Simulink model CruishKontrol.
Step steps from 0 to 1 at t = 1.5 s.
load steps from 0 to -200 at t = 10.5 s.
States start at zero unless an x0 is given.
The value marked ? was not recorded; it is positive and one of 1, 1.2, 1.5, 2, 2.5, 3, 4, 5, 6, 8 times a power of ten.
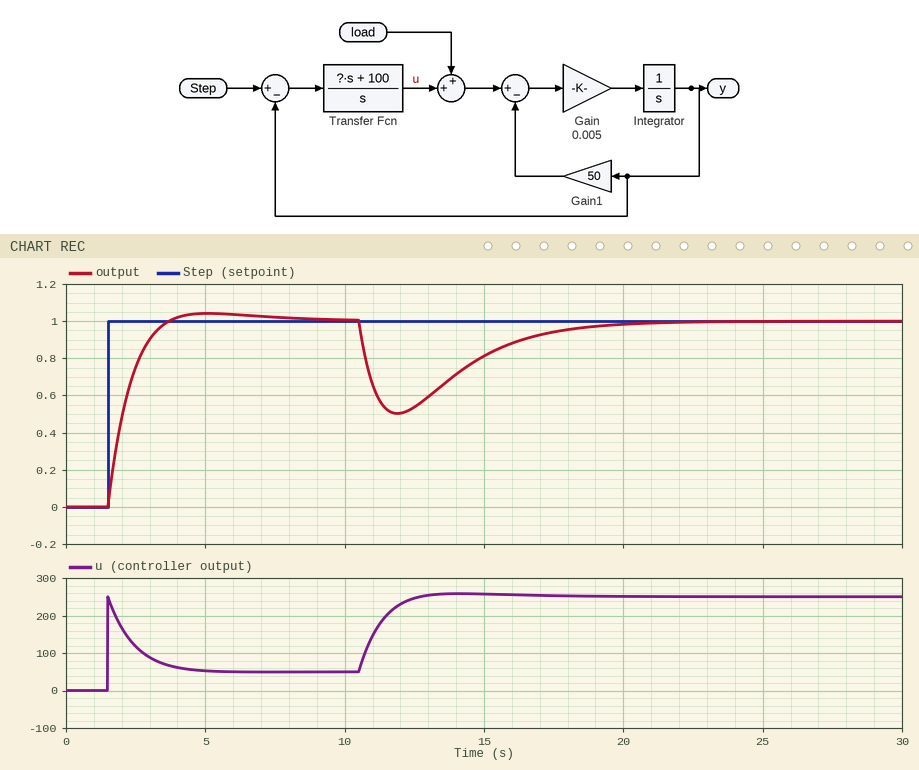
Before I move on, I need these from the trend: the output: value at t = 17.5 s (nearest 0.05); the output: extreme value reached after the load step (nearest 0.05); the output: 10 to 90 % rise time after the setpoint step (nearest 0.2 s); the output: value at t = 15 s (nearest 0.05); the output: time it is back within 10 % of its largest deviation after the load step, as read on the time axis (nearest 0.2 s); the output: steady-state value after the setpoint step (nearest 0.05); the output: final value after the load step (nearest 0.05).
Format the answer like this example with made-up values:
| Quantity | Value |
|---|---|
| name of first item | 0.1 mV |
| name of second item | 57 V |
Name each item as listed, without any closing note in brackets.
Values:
| Quantity | Value |
|---|---|
| the output: value at t = 17.5 s | 0.95 |
| the output: extreme value reached after the load step | 0.50 |
| the output: 10 to 90 % rise time after the setpoint step | 1.4 s |
| the output: value at t = 15 s | 0.80 |
| the output: time it is back within 10 % of its largest deviation after the load step, as read on the time axis | 17.8 s |
| the output: steady-state value after the setpoint step | 1.00 |
| the output: final value after the load step | 1.00 |
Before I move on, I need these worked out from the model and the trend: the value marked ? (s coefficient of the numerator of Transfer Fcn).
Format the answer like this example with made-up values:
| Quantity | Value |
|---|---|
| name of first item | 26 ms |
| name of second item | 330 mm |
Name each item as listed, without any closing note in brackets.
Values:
| Quantity | Value |
|---|---|
| the value marked ? | 250 |
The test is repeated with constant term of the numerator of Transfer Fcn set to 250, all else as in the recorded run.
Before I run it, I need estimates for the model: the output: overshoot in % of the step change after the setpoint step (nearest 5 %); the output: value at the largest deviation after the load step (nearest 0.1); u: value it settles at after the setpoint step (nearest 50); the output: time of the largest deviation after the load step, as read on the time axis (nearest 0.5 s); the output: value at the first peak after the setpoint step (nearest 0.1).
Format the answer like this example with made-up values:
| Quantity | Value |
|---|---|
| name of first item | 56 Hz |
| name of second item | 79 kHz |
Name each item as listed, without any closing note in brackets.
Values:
| Quantity | Value |
|---|---|
| the output: overshoot in % of the step change after the setpoint step | 15 % |
| the output: value at the largest deviation after the load step | 0.6 |
| u: value it settles at after the setpoint step | 50 |
| the output: time of the largest deviation after the load step, as read on the time axis | 11.5 s |
| the output: value at the first peak after the setpoint step | 1.2 |
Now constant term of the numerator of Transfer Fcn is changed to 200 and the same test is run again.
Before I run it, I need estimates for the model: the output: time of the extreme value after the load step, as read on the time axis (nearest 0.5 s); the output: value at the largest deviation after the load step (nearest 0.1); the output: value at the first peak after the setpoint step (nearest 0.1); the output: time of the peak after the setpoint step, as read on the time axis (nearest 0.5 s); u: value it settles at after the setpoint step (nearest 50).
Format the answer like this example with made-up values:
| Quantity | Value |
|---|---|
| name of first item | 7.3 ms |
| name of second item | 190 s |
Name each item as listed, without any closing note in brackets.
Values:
| Quantity | Value |
|---|---|
| the output: time of the extreme value after the load step, as read on the time axis | 11.5 s |
| the output: value at the largest deviation after the load step | 0.6 |
| the output: value at the first peak after the setpoint step | 1.1 |
| the output: time of the peak after the setpoint step, as read on the time axis | 4.0 s |
| u: value it settles at after the setpoint step | 50 |
